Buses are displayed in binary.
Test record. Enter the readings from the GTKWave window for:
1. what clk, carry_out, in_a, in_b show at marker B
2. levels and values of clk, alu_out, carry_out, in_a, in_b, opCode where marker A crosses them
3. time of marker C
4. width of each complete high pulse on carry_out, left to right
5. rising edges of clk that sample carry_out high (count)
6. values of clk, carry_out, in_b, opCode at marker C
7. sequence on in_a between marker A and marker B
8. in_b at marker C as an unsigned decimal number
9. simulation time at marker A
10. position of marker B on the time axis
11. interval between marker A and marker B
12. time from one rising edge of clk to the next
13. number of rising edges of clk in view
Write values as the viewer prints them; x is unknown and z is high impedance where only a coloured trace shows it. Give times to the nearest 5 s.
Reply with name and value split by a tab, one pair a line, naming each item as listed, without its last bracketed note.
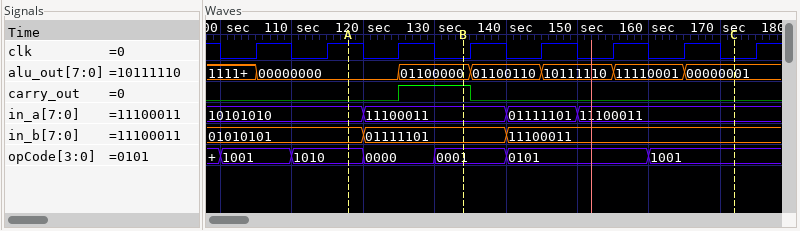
what clk, carry_out, in_a, in_b show at marker B	clk=0, carry_out=1, in_a=11100011, in_b=01111101
levels and values of clk, alu_out, carry_out, in_a, in_b, opCode where marker A crosses them	clk=1, alu_out=00000000, carry_out=0, in_a=10101010, in_b=01010101, opCode=1010
time of marker C	170 s
width of each complete high pulse on carry_out, left to right	10 s
rising edges of clk that sample carry_out high	1
values of clk, carry_out, in_b, opCode at marker C	clk=0, carry_out=0, in_b=11100011, opCode=1001
sequence on in_a between marker A and marker B	10101010, 11100011
in_b at marker C as an unsigned decimal number	227
simulation time at marker A	120 s
position of marker B on the time axis	135 s
interval between marker A and marker B	15 s
time from one rising edge of clk to the next	10 s
number of rising edges of clk in view	8
